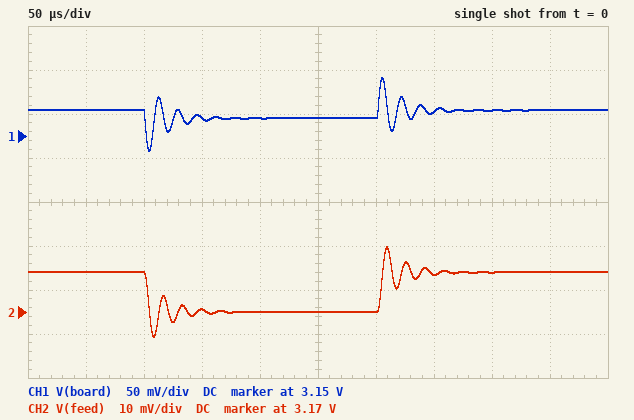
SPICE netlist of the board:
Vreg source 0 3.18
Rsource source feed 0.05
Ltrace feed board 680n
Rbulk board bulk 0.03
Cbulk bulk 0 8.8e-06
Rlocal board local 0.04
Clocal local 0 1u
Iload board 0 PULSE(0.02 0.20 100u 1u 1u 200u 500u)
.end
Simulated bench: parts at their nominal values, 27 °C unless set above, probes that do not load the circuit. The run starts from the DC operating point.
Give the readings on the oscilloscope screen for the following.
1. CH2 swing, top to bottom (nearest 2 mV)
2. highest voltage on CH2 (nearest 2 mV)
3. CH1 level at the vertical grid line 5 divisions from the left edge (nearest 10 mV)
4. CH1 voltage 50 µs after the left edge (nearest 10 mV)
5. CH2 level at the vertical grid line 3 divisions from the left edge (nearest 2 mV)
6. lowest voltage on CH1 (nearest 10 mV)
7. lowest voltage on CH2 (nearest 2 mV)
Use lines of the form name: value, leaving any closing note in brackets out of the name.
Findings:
CH2 swing, top to bottom: 20 mV
highest voltage on CH2: 3.184 V
CH1 level at the vertical grid line 5 divisions from the left edge: 3.17 V
CH1 voltage 50 µs after the left edge: 3.18 V
CH2 level at the vertical grid line 3 divisions from the left edge: 3.170 V
lowest voltage on CH1: 3.13 V
lowest voltage on CH2: 3.164 V
